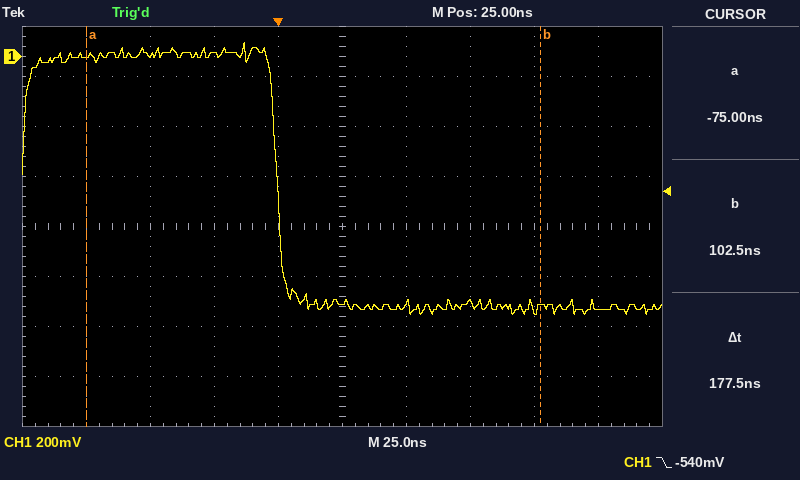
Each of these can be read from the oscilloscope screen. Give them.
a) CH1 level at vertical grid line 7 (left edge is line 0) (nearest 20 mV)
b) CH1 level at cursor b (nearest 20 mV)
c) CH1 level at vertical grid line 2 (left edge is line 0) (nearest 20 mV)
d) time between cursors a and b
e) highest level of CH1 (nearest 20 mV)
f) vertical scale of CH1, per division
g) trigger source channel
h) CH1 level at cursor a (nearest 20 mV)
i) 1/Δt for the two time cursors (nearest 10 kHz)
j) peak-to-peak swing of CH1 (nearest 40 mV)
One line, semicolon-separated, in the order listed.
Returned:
-980 mV; -1.00 V; 0 mV; 177.5 ns; 60 mV; 200 mV; CH1; 0 mV; 5.63 MHz; 1.08 V
